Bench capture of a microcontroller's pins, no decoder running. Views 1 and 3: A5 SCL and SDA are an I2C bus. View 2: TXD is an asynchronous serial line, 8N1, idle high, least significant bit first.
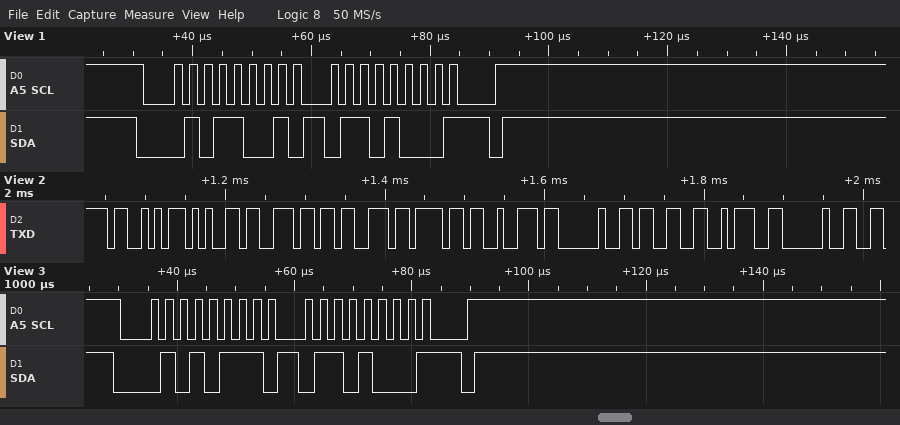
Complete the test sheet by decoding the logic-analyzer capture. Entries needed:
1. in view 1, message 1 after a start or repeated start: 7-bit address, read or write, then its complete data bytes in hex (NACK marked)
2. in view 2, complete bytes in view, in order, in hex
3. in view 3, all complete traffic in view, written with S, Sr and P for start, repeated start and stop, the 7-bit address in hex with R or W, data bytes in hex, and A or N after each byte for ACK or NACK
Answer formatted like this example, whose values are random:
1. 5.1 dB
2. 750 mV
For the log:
1. 0x2C read: 68 NACK
2. 0x53 0x65 0x6E 0x73 0x6F 0x72 0x20 0x33 0x3A 0x20
3. S 2BR A 68 N P
